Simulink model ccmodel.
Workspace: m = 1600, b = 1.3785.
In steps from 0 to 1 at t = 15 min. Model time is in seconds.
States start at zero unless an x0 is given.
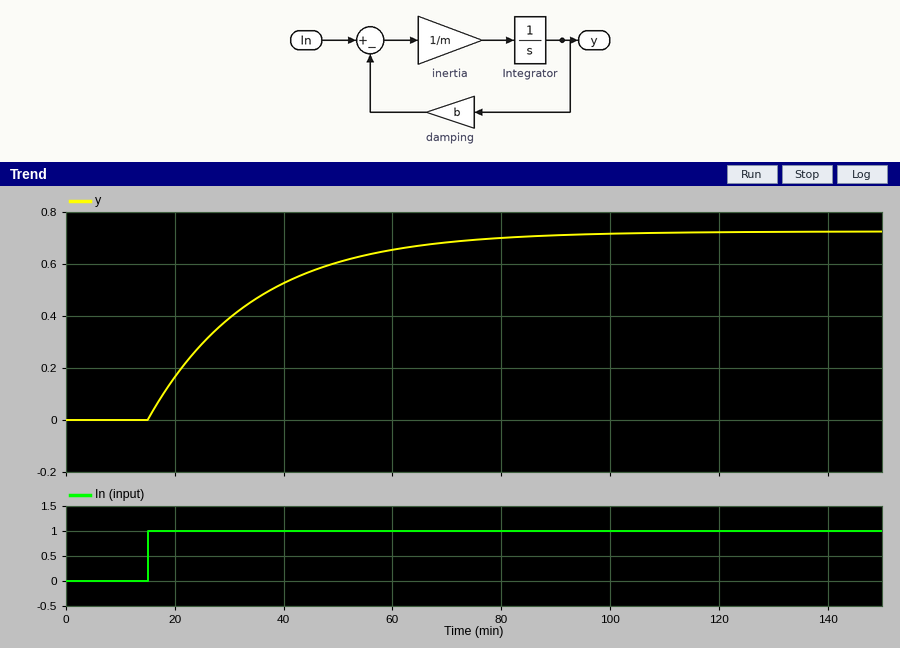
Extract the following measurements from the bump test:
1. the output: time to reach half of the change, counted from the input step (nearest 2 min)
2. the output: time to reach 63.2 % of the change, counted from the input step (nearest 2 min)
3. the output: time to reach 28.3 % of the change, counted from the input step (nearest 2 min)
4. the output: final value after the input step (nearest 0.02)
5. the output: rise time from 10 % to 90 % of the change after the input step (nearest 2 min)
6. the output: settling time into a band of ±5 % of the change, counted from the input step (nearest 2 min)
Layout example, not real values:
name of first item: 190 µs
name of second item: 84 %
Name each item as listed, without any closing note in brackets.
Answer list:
the output: time to reach half of the change, counted from the input step: 14 min
the output: time to reach 63.2 % of the change, counted from the input step: 20 min
the output: time to reach 28.3 % of the change, counted from the input step: 6 min
the output: final value after the input step: 0.72
the output: rise time from 10 % to 90 % of the change after the input step: 42 min
the output: settling time into a band of ±5 % of the change, counted from the input step: 58 min
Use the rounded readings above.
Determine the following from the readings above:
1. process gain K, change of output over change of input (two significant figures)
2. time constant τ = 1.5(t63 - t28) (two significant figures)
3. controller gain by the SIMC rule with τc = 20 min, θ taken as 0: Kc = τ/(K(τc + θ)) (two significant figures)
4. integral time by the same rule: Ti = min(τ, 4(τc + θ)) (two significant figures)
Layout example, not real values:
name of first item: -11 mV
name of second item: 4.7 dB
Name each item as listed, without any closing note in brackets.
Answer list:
process gain K, change of output over change of input: 0.72
time constant τ = 1.5(t63 - t28): 21 min
controller gain by the SIMC rule with τc = 20 min, θ taken as 0: Kc = τ/(K(τc + θ)): 1.5
integral time by the same rule: Ti = min(τ, 4(τc + θ)): 21 min
